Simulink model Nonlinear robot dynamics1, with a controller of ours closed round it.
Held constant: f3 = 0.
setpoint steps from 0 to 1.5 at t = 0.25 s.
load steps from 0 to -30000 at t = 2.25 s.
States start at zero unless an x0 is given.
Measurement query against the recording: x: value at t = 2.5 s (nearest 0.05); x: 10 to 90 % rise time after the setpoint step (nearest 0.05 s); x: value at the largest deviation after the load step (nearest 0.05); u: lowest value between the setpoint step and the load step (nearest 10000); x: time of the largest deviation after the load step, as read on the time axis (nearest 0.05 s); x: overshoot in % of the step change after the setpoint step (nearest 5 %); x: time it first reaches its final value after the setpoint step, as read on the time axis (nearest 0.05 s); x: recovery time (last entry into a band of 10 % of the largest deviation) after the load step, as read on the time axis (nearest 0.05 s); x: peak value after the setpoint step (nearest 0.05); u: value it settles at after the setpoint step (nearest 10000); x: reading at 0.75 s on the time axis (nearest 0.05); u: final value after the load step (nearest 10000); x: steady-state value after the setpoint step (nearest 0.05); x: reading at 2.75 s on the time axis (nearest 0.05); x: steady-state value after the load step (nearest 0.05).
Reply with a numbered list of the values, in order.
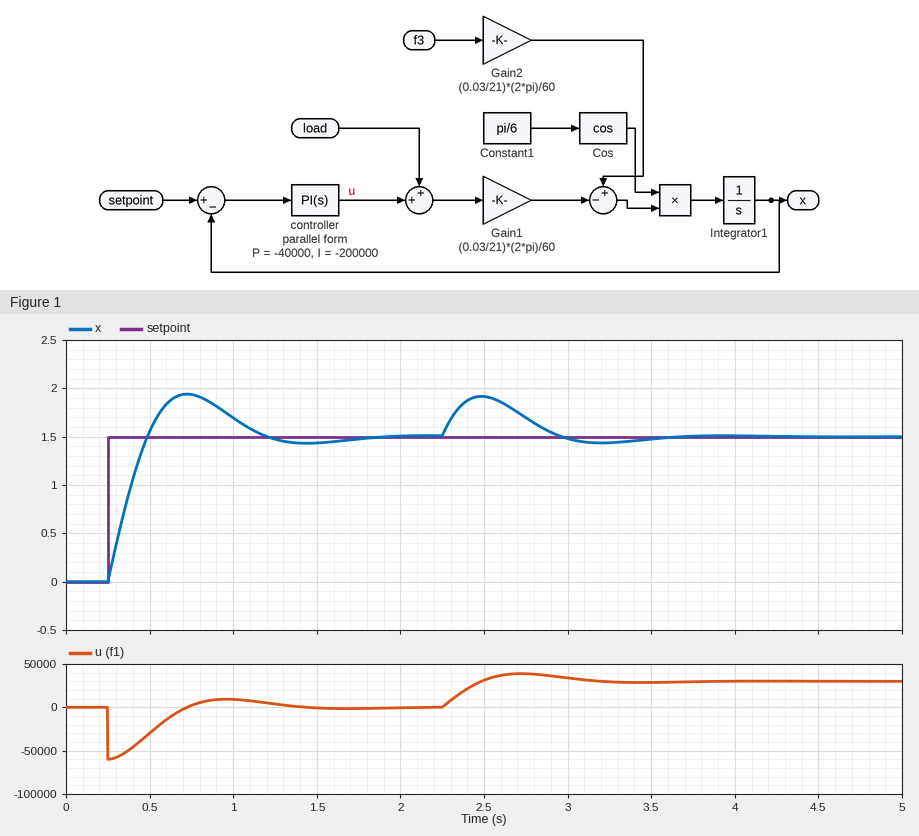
1. 1.90
2. 0.20 s
3. 1.90
4. -60000
5. 2.50 s
6. 30 %
7. 0.50 s
8. 3.40 s
9. 1.95
10. 0
11. 1.95
12. 30000
13. 1.50
14. 1.70
15. 1.50
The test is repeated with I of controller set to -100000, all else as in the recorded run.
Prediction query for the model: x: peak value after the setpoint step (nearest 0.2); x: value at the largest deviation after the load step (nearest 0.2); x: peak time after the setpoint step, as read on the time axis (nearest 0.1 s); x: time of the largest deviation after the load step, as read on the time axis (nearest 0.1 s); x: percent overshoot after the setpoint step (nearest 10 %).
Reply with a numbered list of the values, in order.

1. 1.8
2. 2.0
3. 0.9 s
4. 2.6 s
5. 20 %
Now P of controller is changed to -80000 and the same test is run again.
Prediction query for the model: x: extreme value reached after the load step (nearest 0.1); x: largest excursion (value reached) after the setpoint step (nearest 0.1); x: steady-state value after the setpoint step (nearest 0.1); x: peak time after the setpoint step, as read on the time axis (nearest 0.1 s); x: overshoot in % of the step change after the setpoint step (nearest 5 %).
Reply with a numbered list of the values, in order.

1. 1.8
2. 1.7
3. 1.5
4. 0.6 s
5. 15 %
